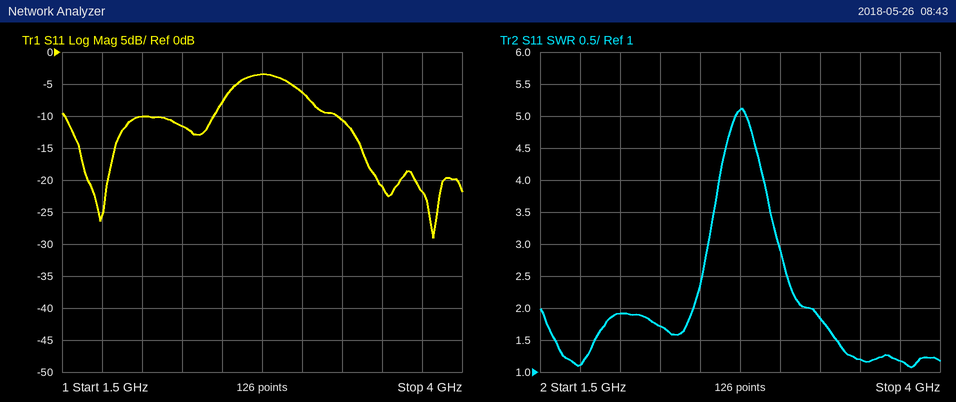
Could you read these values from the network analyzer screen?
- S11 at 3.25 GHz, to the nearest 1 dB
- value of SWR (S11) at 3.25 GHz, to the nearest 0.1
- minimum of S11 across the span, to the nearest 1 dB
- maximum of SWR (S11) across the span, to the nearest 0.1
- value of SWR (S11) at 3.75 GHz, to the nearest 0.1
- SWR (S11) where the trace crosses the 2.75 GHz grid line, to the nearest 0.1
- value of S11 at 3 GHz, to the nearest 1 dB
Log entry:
-11 dB
1.8
-29 dB
5.1
1.2
5.1
-6 dB
